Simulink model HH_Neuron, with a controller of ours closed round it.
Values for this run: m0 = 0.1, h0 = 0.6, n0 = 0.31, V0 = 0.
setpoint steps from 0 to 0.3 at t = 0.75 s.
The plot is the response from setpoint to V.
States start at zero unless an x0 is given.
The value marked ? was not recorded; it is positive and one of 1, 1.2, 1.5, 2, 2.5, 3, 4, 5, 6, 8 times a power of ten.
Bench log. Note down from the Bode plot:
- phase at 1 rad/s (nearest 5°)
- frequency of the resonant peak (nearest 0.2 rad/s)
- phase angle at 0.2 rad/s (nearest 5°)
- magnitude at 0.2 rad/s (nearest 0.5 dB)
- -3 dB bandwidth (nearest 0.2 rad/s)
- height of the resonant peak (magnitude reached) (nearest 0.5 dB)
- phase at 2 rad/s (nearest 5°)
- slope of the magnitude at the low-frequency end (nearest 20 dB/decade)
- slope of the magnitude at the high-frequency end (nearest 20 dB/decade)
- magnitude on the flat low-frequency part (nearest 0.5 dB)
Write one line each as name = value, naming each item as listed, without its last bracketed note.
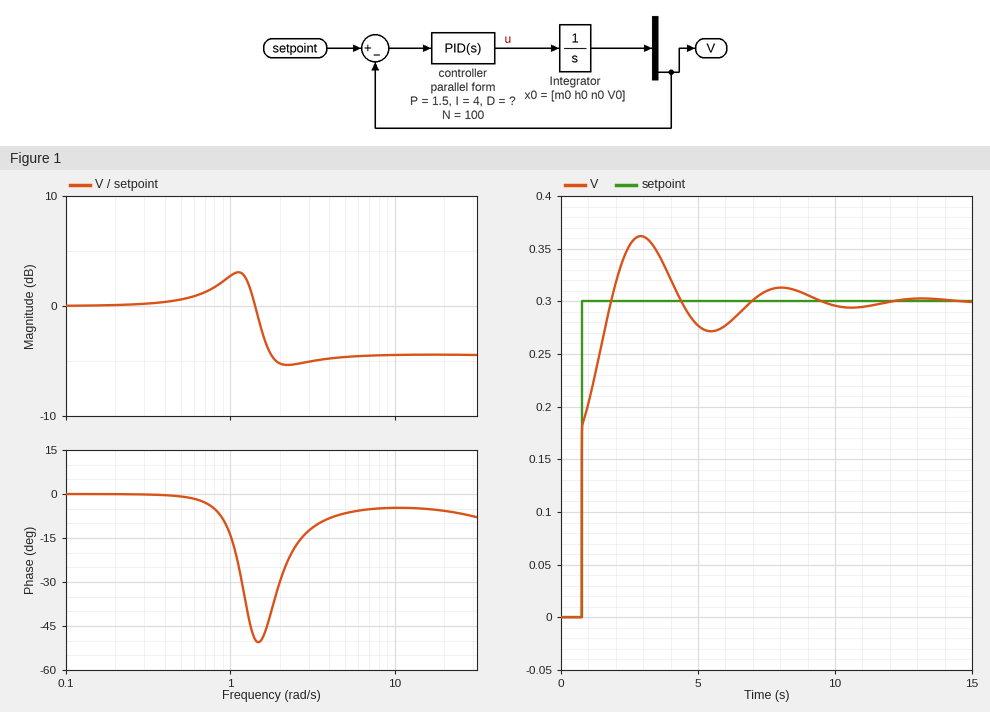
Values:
phase at 1 rad/s = -15°
frequency of the resonant peak = 1.2 rad/s
phase angle at 0.2 rad/s = 0°
magnitude at 0.2 rad/s = 0.0 dB
-3 dB bandwidth = 1.6 rad/s
height of the resonant peak (magnitude reached) = 3.0 dB
phase at 2 rad/s = -30°
slope of the magnitude at the low-frequency end = 0 dB/decade
slope of the magnitude at the high-frequency end = 0 dB/decade
magnitude on the flat low-frequency part = 0.0 dB
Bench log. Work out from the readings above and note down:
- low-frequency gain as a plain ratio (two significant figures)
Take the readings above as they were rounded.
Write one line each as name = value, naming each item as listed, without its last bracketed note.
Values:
low-frequency gain as a plain ratio = 1.0
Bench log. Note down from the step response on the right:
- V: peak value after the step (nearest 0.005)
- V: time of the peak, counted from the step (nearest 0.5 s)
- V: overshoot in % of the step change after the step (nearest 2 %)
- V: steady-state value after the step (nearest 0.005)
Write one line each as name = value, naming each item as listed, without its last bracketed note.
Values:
V: peak value after the step = 0.360
V: time of the peak, counted from the step = 2.0 s
V: overshoot in % of the step change after the step = 20 %
V: steady-state value after the step = 0.300
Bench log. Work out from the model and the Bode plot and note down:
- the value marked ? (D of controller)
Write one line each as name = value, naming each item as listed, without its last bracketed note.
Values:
the value marked ? = 1.5
